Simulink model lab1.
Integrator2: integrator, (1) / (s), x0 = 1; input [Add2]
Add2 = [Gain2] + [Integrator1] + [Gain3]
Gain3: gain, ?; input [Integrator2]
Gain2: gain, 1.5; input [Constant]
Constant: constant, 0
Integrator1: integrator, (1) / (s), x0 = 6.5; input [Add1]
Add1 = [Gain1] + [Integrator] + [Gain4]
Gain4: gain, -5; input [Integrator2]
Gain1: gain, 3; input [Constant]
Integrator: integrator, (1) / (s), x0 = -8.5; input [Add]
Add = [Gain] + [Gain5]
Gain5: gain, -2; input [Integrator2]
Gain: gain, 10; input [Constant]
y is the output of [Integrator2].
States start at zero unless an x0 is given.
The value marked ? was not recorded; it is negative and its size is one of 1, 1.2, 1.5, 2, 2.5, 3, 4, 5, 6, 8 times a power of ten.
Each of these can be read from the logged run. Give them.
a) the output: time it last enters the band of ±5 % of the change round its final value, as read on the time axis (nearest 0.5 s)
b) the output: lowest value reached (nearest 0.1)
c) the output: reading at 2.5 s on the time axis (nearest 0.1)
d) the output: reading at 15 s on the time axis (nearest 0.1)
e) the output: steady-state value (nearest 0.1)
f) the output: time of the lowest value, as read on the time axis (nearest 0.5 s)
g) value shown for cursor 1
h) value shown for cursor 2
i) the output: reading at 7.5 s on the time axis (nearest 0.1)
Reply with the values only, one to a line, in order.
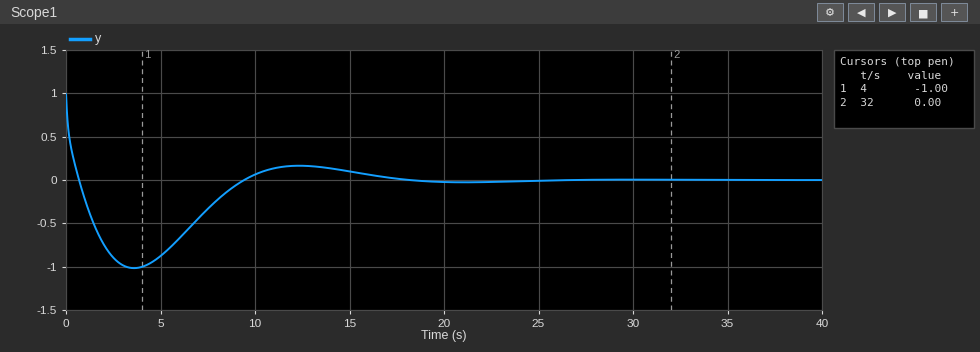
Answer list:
16.5 s
-1.0
-0.9
0.1
0.0
3.5 s
-1.00
0.00
-0.3
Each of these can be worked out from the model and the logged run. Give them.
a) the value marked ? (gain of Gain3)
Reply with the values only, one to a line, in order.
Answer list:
-12
